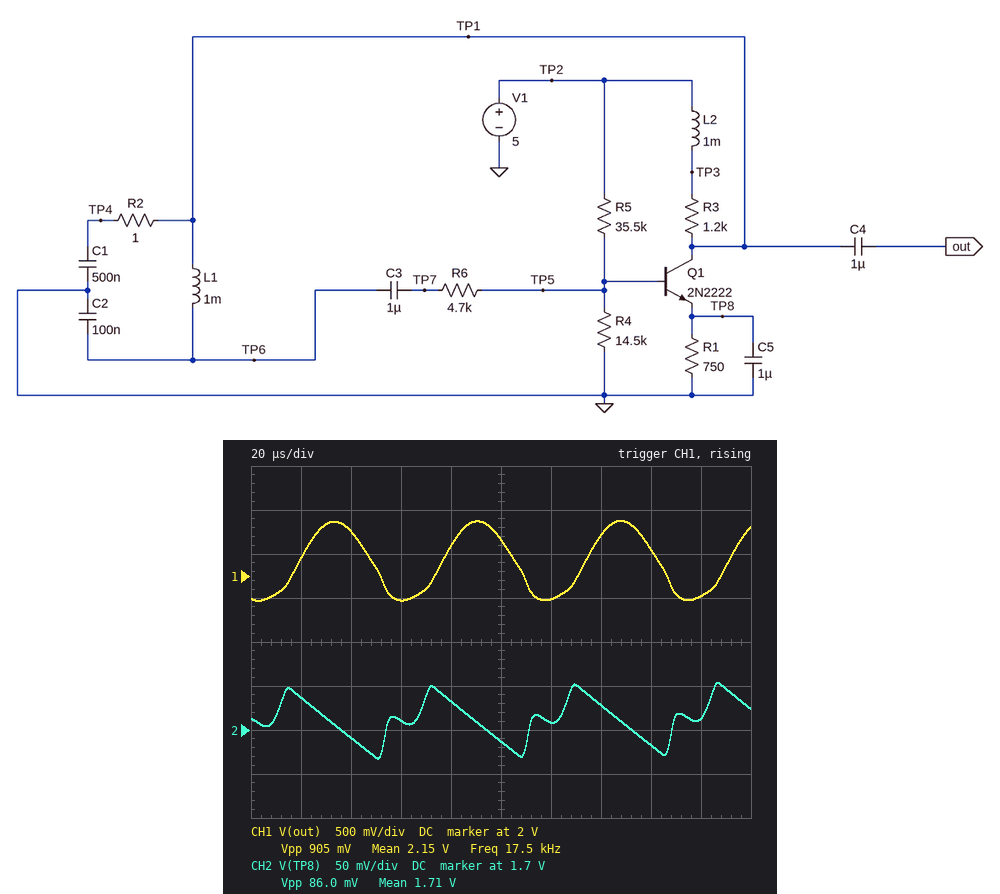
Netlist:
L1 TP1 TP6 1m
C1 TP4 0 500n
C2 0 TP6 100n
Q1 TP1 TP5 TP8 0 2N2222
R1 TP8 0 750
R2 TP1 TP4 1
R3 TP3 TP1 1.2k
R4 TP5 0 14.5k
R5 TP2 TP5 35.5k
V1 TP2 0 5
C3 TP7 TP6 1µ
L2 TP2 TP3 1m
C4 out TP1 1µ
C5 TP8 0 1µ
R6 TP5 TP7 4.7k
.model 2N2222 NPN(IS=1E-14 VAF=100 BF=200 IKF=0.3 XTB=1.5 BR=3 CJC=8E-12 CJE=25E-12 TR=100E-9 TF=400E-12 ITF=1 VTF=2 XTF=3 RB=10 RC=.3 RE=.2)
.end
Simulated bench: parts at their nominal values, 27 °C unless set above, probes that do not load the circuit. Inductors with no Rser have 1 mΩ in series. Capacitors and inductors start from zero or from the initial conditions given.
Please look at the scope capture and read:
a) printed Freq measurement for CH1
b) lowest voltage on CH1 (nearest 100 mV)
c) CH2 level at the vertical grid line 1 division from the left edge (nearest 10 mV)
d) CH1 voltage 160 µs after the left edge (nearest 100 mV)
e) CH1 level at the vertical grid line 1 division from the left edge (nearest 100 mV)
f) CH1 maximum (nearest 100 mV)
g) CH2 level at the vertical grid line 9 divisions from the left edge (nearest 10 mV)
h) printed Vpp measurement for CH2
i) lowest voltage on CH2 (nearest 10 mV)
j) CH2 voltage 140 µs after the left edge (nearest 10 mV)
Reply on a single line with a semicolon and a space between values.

17.5 kHz; 1.7 V; 1.74 V; 2.3 V; 2.2 V; 2.6 V; 1.71 V; 86.0 mV; 1.67 V; 1.73 V
